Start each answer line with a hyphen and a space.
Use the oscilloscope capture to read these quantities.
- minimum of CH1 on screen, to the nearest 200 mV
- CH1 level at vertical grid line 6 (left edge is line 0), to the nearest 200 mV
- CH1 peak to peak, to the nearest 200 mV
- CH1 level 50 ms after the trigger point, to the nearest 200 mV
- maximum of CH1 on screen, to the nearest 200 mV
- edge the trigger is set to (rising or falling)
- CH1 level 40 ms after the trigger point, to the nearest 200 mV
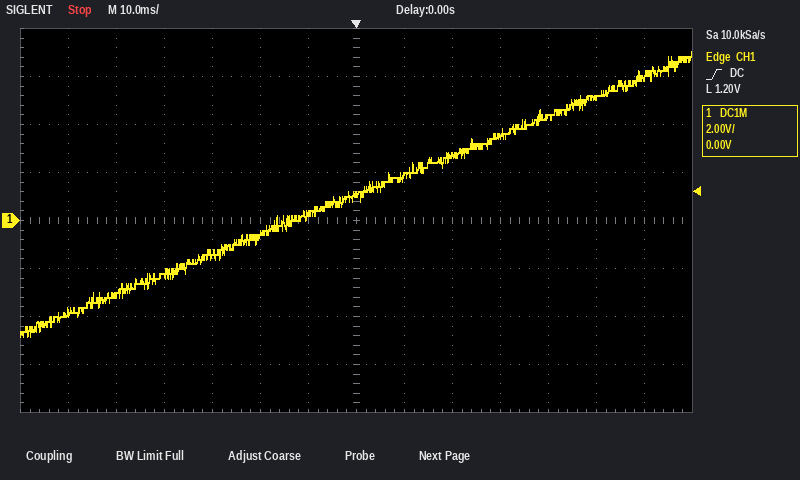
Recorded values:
- -4.8 V
- 200 mV
- 11.8 V
- 5.2 V
- 7.0 V
- rising
- 4.4 V
